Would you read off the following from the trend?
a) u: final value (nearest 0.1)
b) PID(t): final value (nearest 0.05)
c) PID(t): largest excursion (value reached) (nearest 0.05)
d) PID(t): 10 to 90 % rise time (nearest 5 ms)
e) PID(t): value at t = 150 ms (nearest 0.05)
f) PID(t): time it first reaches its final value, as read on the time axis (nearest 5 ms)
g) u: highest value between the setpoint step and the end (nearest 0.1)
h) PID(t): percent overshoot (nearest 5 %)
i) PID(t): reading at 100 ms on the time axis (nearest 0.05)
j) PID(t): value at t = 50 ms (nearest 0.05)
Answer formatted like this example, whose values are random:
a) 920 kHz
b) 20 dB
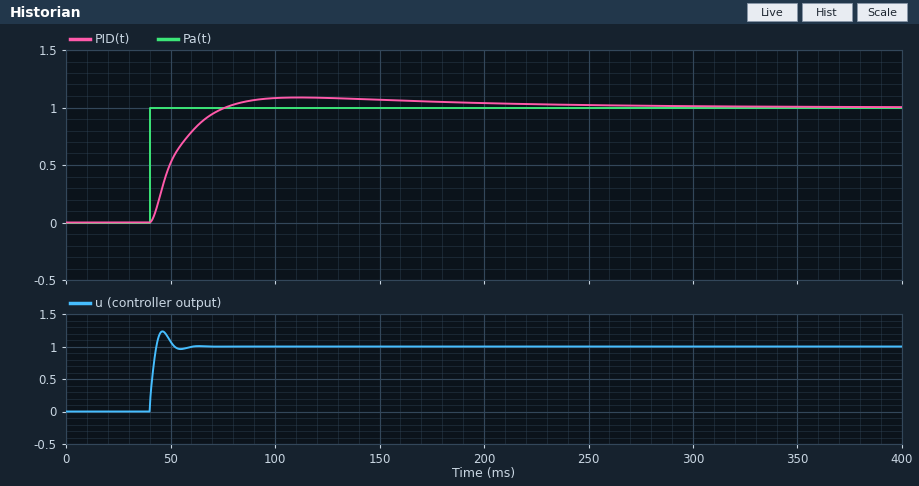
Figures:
a) 1.0
b) 1.00
c) 1.10
d) 25 ms
e) 1.05
f) 75 ms
g) 1.2
h) 10 %
i) 1.10
j) 0.50
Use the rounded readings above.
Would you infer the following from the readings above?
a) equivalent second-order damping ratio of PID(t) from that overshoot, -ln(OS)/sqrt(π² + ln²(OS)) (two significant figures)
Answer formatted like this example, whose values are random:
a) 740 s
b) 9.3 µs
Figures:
a) 0.59
